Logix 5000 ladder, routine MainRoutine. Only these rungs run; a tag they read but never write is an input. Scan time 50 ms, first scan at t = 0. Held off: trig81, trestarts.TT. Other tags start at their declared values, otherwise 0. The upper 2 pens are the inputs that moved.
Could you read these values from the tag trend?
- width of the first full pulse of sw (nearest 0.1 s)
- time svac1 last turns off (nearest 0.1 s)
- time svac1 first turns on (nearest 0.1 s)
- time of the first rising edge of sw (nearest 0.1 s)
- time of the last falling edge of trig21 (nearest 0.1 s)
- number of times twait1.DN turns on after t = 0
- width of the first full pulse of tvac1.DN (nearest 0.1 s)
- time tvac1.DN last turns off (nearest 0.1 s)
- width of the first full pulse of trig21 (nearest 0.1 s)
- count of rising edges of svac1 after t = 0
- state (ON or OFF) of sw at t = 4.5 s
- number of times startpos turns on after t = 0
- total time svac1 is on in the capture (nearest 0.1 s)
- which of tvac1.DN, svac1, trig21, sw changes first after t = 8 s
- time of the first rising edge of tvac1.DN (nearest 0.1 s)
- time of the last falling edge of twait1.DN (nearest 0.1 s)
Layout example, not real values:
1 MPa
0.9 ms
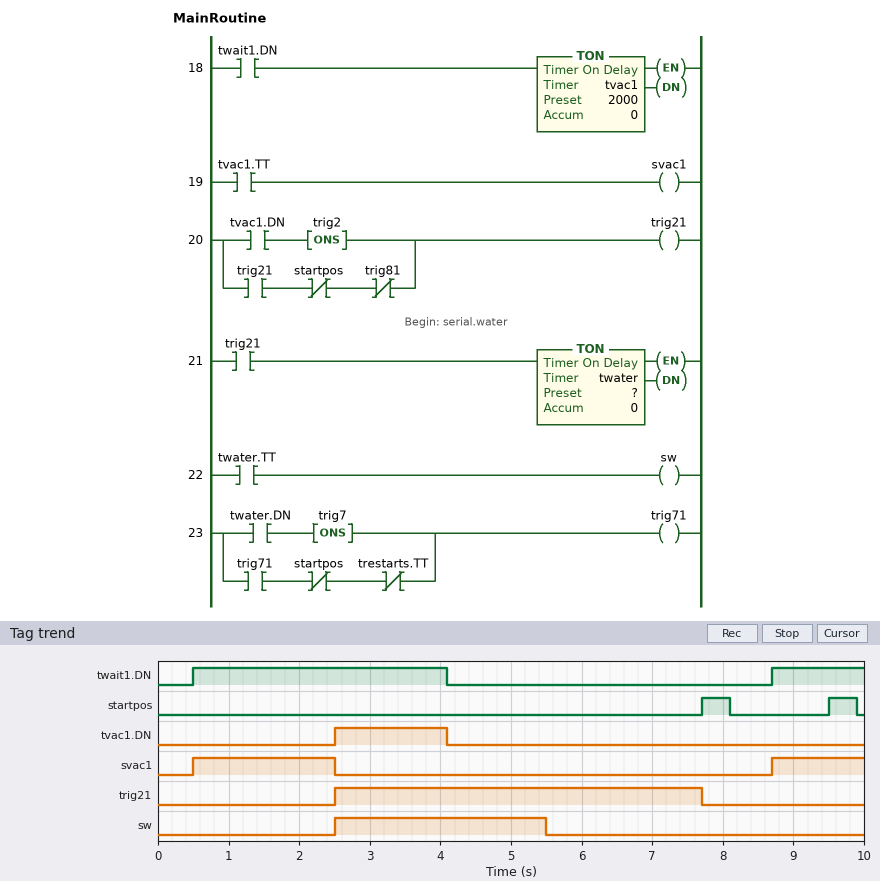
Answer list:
3.0 s
2.5 s
0.5 s
2.5 s
7.7 s
2
1.6 s
4.1 s
5.2 s
2
ON
2
3.3 s
svac1
2.5 s
4.1 s
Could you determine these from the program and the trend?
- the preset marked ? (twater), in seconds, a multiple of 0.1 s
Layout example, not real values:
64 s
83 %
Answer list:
3.0 s
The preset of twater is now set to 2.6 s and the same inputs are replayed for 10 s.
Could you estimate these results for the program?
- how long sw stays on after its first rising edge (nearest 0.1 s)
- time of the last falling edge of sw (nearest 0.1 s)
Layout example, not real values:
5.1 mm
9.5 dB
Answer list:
2.6 s
5.1 s
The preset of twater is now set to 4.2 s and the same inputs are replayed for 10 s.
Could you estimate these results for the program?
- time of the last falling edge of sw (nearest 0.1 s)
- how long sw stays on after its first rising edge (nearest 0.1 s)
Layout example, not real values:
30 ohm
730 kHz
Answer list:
6.7 s
4.2 s
